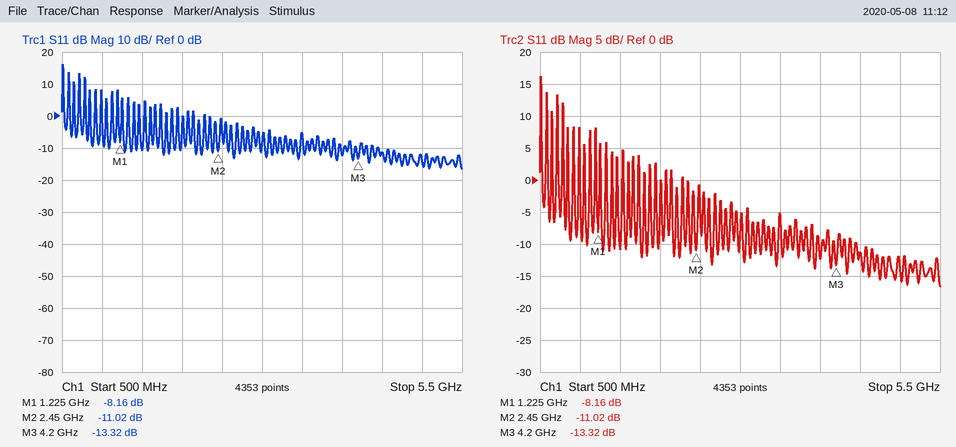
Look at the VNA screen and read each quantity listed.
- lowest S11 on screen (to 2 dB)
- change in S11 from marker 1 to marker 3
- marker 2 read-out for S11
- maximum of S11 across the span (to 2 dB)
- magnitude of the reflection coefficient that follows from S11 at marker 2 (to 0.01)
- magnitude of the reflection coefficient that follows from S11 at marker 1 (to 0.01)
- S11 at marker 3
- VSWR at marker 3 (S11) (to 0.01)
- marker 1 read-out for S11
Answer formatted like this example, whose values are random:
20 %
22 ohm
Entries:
-16 dB
-5.16 dB
-11.02 dB
16 dB
0.28
0.39
-13.32 dB
1.55
-8.16 dB
